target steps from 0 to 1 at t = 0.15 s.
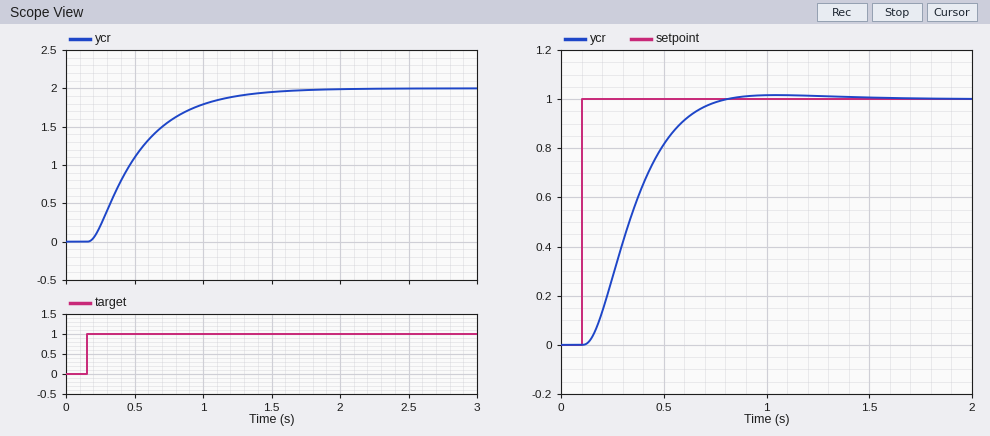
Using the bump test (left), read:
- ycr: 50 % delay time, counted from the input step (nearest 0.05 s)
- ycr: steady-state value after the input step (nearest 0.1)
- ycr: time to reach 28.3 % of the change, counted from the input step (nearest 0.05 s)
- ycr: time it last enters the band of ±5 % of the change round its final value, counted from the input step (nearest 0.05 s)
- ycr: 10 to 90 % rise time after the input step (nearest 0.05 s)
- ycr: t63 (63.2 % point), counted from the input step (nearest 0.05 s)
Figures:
0.30 s
2.0
0.20 s
1.10 s
0.75 s
0.40 s
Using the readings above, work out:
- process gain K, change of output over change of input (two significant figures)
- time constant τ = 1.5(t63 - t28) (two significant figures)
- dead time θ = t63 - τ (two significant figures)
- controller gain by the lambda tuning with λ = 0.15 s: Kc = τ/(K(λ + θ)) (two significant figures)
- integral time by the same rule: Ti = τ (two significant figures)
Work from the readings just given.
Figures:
2.0
0.30 s
0.10 s
0.60
0.30 s
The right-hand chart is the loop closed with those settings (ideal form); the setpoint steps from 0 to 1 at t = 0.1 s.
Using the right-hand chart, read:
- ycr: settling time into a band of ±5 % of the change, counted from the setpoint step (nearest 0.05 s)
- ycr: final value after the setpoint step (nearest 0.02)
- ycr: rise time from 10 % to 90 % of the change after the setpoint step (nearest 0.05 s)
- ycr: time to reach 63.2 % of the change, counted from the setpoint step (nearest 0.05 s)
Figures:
0.55 s
1.00
0.40 s
0.30 s
